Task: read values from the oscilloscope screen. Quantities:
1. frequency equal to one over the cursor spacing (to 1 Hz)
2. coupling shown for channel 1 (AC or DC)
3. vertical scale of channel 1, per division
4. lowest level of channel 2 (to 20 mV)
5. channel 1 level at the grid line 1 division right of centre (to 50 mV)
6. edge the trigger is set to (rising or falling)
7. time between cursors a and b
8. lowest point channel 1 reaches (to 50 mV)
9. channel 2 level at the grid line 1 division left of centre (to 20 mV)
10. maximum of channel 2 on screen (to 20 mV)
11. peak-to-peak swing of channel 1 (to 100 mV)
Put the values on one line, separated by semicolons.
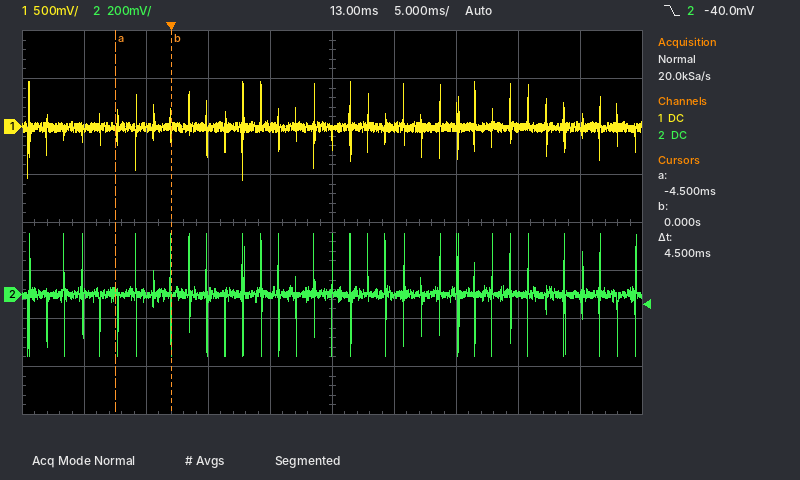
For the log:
222 Hz; DC; 500 mV; -260 mV; 0 mV; falling; 4.5 ms; -550 mV; 0 mV; 260 mV; 1.00 V
